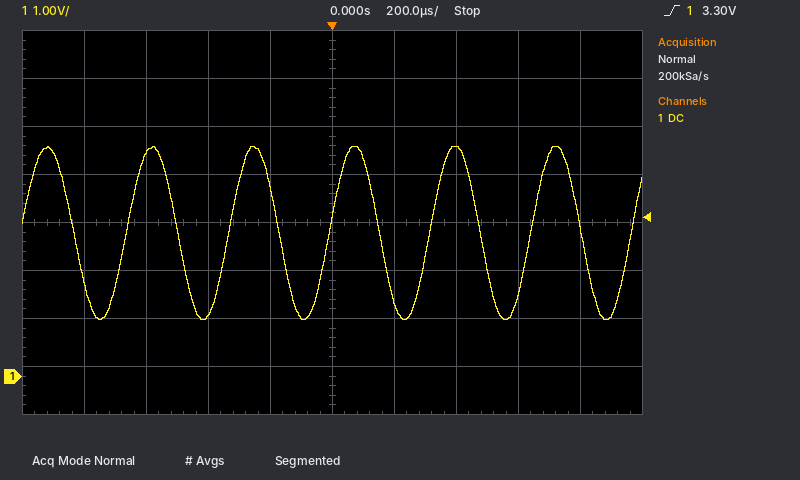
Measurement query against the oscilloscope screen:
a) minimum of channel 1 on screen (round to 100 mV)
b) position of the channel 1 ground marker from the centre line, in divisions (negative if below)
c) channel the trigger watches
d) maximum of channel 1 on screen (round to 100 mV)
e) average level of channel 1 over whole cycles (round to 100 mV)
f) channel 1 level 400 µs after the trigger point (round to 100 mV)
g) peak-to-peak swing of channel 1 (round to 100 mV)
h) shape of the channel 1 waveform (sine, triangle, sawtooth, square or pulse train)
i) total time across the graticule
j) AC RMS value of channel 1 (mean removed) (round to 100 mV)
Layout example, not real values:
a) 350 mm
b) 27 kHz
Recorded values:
a) 1.2 V
b) -3.2 div
c) channel 1
d) 4.8 V
e) 3.0 V
f) 4.8 V
g) 3.6 V
h) sine
i) 2 ms
j) 1.3 V
